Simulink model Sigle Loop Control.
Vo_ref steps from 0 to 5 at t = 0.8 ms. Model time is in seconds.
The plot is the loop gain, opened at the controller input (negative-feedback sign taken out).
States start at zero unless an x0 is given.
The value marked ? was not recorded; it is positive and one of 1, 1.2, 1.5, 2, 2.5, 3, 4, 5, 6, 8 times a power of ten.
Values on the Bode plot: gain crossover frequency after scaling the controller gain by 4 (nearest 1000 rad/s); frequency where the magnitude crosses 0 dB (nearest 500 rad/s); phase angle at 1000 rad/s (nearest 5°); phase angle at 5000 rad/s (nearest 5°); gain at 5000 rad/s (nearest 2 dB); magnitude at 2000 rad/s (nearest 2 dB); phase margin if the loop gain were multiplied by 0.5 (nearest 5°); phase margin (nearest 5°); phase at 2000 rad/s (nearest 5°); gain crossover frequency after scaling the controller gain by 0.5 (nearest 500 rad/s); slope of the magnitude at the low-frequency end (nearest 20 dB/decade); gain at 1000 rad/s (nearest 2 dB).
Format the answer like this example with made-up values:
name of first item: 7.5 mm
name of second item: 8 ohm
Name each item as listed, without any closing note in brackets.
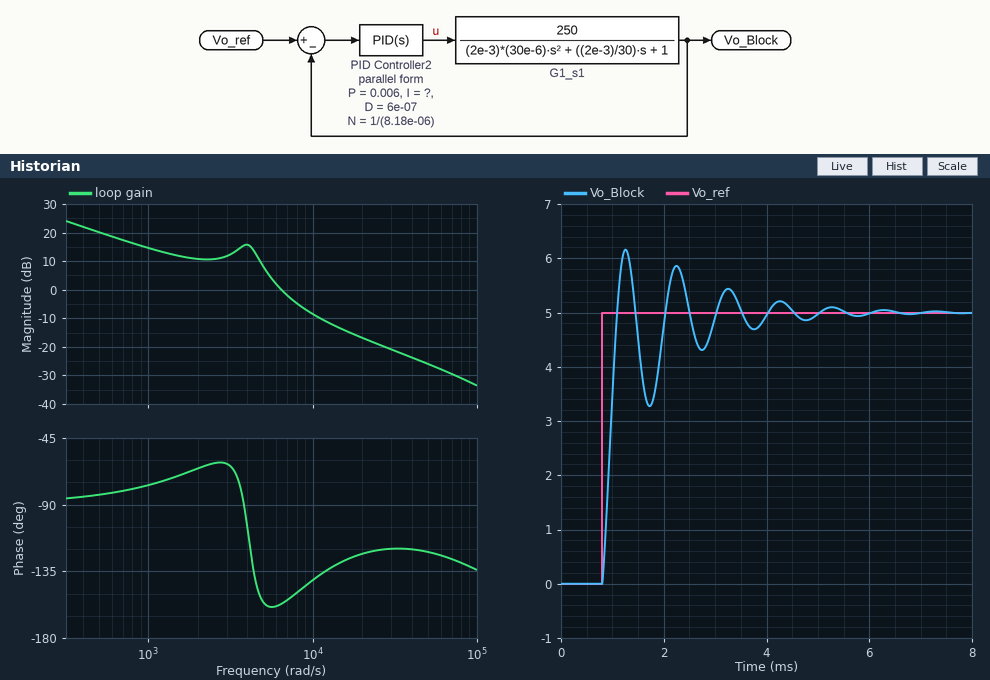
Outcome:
gain crossover frequency after scaling the controller gain by 4: 13000 rad/s
frequency where the magnitude crosses 0 dB: 6500 rad/s
phase angle at 1000 rad/s: -75°
phase angle at 5000 rad/s: -155°
gain at 5000 rad/s: 8 dB
magnitude at 2000 rad/s: 10 dB
phase margin if the loop gain were multiplied by 0.5: 20°
phase margin: 25°
phase at 2000 rad/s: -65°
gain crossover frequency after scaling the controller gain by 0.5: 5500 rad/s
slope of the magnitude at the low-frequency end: -20 dB/decade
gain at 1000 rad/s: 14 dB
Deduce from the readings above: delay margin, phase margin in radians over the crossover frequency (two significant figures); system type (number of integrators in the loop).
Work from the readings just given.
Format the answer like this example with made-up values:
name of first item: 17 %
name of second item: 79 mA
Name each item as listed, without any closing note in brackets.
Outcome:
delay margin, phase margin in radians over the crossover frequency: 0.000067 s
system type: 1
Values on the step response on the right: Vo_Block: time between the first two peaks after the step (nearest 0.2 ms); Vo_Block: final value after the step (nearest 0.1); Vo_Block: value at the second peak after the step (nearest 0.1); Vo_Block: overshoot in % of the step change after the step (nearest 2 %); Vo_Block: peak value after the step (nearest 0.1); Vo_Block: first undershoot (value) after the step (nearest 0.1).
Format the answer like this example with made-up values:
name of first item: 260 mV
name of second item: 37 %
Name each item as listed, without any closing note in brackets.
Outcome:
Vo_Block: time between the first two peaks after the step: 1.0 ms
Vo_Block: final value after the step: 5.0
Vo_Block: value at the second peak after the step: 5.9
Vo_Block: overshoot in % of the step change after the step: 24 %
Vo_Block: peak value after the step: 6.2
Vo_Block: first undershoot (value) after the step: 3.3
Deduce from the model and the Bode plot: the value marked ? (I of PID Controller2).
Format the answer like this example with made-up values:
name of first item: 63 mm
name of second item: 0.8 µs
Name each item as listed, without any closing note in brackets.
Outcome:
the value marked ?: 20
